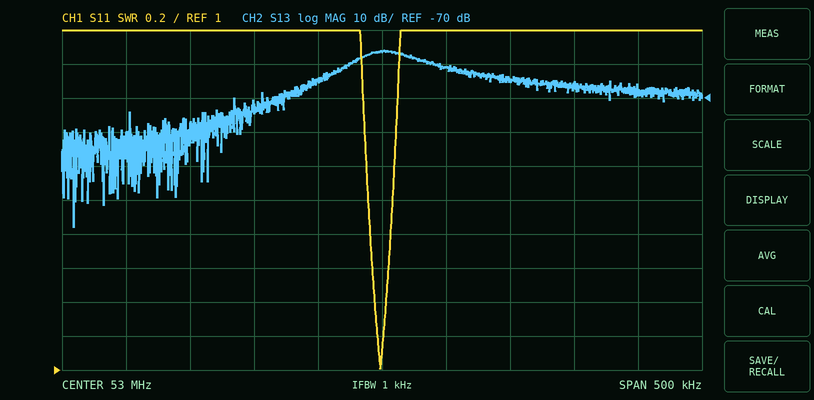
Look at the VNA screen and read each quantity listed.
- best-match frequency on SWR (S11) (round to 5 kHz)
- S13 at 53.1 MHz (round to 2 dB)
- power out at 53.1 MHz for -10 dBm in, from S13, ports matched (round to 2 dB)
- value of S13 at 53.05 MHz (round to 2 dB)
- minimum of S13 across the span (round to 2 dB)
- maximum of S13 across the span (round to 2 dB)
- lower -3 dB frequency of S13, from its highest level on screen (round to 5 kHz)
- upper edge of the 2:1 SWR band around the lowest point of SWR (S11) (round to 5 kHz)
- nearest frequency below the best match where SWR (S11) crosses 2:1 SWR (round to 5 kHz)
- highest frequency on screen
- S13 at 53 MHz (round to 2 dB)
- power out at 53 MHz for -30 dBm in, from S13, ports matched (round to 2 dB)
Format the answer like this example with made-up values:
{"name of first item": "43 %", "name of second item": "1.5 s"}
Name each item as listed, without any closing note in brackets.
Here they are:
{"best-match frequency on SWR (S11)": "53.000 MHz", "S13 at 53.1 MHz": "-64 dB", "power out at 53.1 MHz for -10 dBm in, from S13, ports matched": "-74 dBm", "value of S13 at 53.05 MHz": "-60 dB", "minimum of S13 across the span": "-108 dB", "maximum of S13 across the span": "-56 dB", "lower -3 dB frequency of S13, from its highest level on screen": "52.980 MHz", "upper edge of the 2:1 SWR band around the lowest point of SWR (S11)": "53.010 MHz", "nearest frequency below the best match where SWR (S11) crosses 2:1 SWR": "52.990 MHz", "highest frequency on screen": "53.25 MHz", "S13 at 53 MHz": "-56 dB", "power out at 53 MHz for -30 dBm in, from S13, ports matched": "-86 dBm"}
